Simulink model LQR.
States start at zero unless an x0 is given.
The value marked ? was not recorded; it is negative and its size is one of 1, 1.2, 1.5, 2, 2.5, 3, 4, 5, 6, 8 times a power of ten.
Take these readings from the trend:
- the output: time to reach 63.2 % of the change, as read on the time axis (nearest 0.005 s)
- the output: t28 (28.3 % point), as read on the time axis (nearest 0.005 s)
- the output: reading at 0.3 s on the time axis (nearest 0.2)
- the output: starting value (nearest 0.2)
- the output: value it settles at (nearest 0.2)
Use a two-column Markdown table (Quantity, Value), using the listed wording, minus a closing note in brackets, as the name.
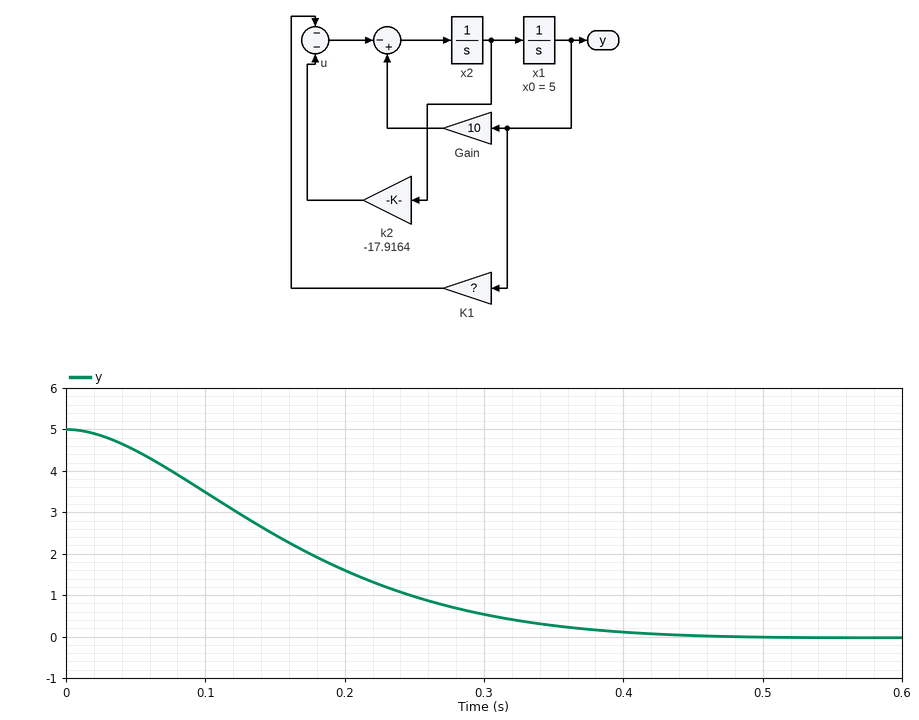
| Quantity | Value |
|---|---|
| the output: time to reach 63.2 % of the change, as read on the time axis | 0.185 s |
| the output: t28 (28.3 % point), as read on the time axis | 0.095 s |
| the output: reading at 0.3 s on the time axis | 0.6 |
| the output: starting value | 5.0 |
| the output: value it settles at | 0.0 |
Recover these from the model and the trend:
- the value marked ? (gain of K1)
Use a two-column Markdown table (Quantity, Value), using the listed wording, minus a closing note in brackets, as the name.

| Quantity | Value |
|---|---|
| the value marked ? | -120 |
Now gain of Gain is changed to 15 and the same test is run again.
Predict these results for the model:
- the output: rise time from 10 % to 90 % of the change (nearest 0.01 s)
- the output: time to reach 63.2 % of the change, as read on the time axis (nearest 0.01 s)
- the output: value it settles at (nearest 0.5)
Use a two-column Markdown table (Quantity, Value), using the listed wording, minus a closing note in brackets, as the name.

| Quantity | Value |
|---|---|
| the output: rise time from 10 % to 90 % of the change | 0.27 s |
| the output: time to reach 63.2 % of the change, as read on the time axis | 0.19 s |
| the output: value it settles at | 0.0 |
